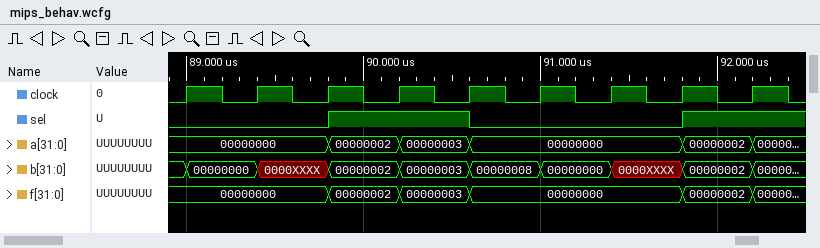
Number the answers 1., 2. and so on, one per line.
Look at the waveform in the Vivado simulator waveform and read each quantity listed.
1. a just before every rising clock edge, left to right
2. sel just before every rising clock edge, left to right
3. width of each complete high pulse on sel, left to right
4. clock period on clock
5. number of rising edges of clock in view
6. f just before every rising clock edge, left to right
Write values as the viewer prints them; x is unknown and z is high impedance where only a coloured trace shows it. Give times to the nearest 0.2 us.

1. 00000000, 00000000, 00000000, 00000002, 00000003, 00000000, 00000000, 00000000, 00000002
2. 0 0 0 1 1 0 0 0 1
3. 0.8 us
4. 0.4 us
5. 9
6. 00000000, 00000000, 00000000, 00000002, 00000003, 00000000, 00000000, 00000000, 00000002
